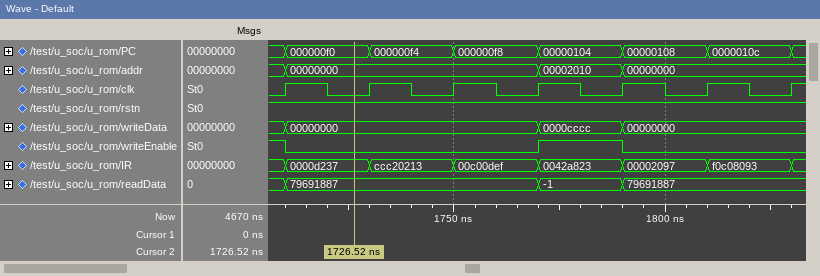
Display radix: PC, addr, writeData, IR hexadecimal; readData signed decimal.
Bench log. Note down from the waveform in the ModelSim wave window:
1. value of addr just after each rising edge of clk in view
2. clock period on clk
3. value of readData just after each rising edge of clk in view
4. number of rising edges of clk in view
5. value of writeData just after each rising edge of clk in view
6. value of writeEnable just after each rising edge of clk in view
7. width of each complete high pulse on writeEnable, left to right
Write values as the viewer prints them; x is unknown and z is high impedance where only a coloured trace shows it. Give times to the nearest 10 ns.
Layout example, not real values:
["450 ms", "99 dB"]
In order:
["00000000, 00000000, 00000000, 00002010, 00000000, 00000000, 00000000", "20 ns", "79691887, 79691887, 79691887, -1, 79691887, 79691887, 79691887", "7", "00000000, 00000000, 00000000, 0000cccc, 00000000, 00000000, 00000000", "0 0 0 1 0 0 0", "20 ns"]
